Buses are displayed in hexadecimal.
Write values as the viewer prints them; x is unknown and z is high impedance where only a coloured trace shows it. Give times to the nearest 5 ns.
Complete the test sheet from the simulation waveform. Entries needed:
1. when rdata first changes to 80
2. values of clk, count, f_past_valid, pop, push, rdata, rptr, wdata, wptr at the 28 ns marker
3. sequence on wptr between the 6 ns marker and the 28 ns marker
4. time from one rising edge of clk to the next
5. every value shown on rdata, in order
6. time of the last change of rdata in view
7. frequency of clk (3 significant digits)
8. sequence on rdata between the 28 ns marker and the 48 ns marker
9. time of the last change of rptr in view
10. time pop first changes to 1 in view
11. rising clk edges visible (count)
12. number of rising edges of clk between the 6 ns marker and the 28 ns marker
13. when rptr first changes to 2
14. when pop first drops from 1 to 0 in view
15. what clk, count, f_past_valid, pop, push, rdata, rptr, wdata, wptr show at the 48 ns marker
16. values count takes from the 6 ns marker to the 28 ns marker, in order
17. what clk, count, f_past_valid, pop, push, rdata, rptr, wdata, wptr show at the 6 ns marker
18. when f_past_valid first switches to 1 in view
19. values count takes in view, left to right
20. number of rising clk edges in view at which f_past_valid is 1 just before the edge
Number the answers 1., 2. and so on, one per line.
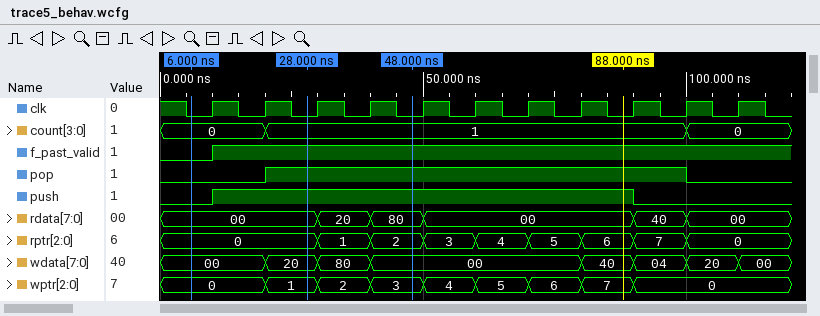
1. 40 ns
2. clk=0, count=1, f_past_valid=1, pop=1, push=1, rdata=00, rptr=0, wdata=20, wptr=1
3. 0, 1
4. 10 ns
5. 00, 20, 80, 00, 40, 00
6. 100 ns
7. 100 MHz
8. 00, 20, 80
9. 100 ns
10. 20 ns
11. 11
12. 2
13. 40 ns
14. 100 ns
15. clk=0, count=1, f_past_valid=1, pop=1, push=1, rdata=80, rptr=2, wdata=00, wptr=3
16. 0, 1
17. clk=0, count=0, f_past_valid=0, pop=0, push=0, rdata=00, rptr=0, wdata=00, wptr=0
18. 10 ns
19. 0, 1, 0
20. 10
